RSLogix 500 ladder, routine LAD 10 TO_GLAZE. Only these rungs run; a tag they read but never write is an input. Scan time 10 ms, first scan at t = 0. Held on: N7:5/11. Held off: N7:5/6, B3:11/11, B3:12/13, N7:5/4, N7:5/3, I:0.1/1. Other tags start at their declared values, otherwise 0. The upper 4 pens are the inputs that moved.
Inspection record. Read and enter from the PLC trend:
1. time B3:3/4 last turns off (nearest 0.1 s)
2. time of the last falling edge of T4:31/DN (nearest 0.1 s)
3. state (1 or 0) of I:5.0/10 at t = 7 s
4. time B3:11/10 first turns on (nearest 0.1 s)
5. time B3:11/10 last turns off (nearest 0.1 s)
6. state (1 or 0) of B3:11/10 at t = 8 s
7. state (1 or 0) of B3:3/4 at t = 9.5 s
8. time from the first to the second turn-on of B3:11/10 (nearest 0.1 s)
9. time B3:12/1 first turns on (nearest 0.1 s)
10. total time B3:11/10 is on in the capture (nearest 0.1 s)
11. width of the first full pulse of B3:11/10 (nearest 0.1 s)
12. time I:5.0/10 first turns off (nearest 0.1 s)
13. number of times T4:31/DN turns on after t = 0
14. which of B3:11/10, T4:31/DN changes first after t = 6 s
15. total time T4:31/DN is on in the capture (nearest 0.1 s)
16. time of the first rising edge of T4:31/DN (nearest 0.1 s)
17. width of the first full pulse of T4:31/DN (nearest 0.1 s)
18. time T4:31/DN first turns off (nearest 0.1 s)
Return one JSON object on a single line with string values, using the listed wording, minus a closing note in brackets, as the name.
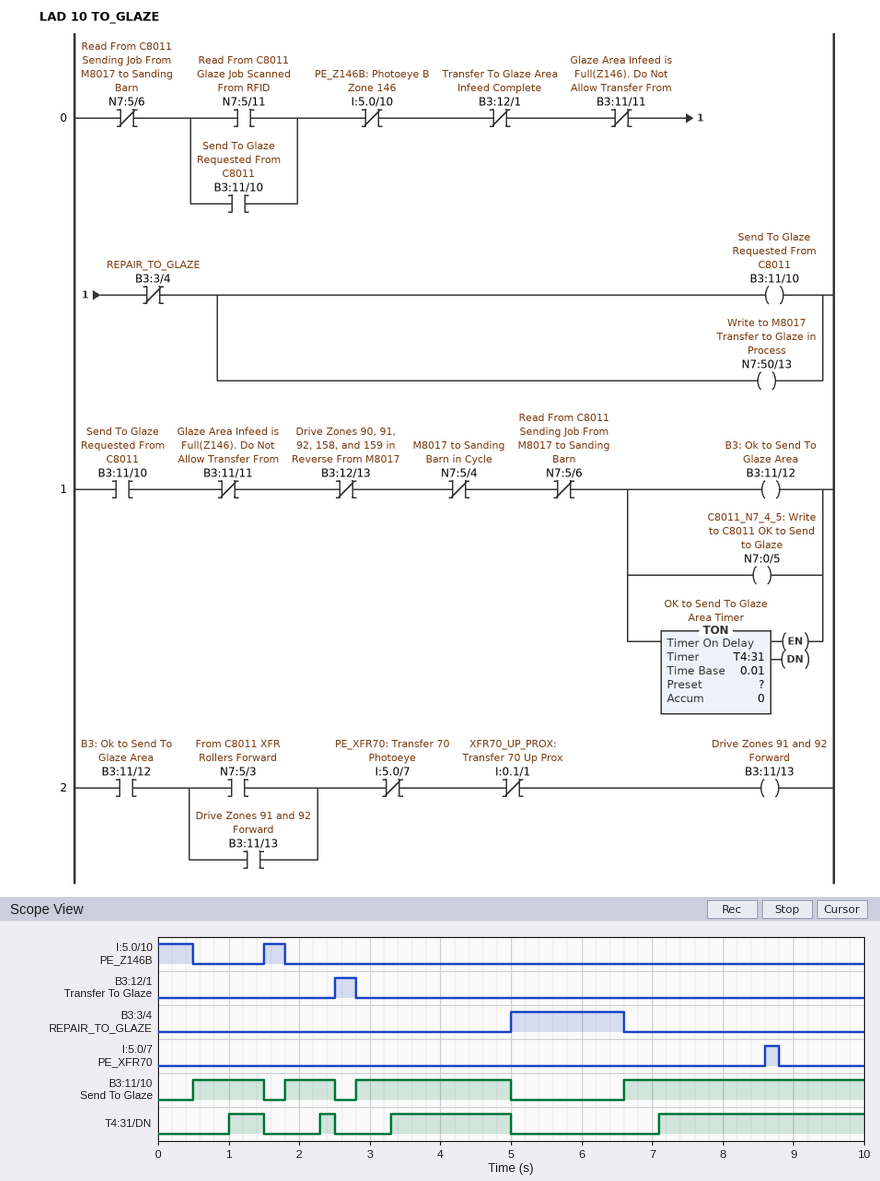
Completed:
{"time B3:3/4 last turns off": "6.6 s", "time of the last falling edge of T4:31/DN": "5.0 s", "state (1 or 0) of I:5.0/10 at t = 7 s": "0", "time B3:11/10 first turns on": "0.5 s", "time B3:11/10 last turns off": "5.0 s", "state (1 or 0) of B3:11/10 at t = 8 s": "1", "state (1 or 0) of B3:3/4 at t = 9.5 s": "0", "time from the first to the second turn-on of B3:11/10": "1.3 s", "time B3:12/1 first turns on": "2.5 s", "total time B3:11/10 is on in the capture": "7.3 s", "width of the first full pulse of B3:11/10": "1.0 s", "time I:5.0/10 first turns off": "0.5 s", "number of times T4:31/DN turns on after t = 0": "4", "which of B3:11/10, T4:31/DN changes first after t = 6 s": "B3:11/10", "total time T4:31/DN is on in the capture": "5.3 s", "time of the first rising edge of T4:31/DN": "1.0 s", "width of the first full pulse of T4:31/DN": "0.5 s", "time T4:31/DN first turns off": "1.5 s"}
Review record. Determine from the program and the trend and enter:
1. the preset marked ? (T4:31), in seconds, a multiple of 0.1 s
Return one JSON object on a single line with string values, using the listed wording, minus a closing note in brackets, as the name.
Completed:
{"the preset marked ? (T4:31), in seconds, a multiple of 0.1 s": "0.5 s"}
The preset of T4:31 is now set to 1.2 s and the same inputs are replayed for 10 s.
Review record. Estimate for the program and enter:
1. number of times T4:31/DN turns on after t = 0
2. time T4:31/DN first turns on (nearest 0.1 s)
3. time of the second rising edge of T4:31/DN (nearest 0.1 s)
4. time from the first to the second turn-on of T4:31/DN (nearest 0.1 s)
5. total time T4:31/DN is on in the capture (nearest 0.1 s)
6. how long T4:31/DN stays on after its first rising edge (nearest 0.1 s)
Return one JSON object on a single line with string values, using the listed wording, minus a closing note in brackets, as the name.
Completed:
{"number of times T4:31/DN turns on after t = 0": "2", "time T4:31/DN first turns on": "4.0 s", "time of the second rising edge of T4:31/DN": "7.8 s", "time from the first to the second turn-on of T4:31/DN": "3.8 s", "total time T4:31/DN is on in the capture": "3.2 s", "how long T4:31/DN stays on after its first rising edge": "1.0 s"}
